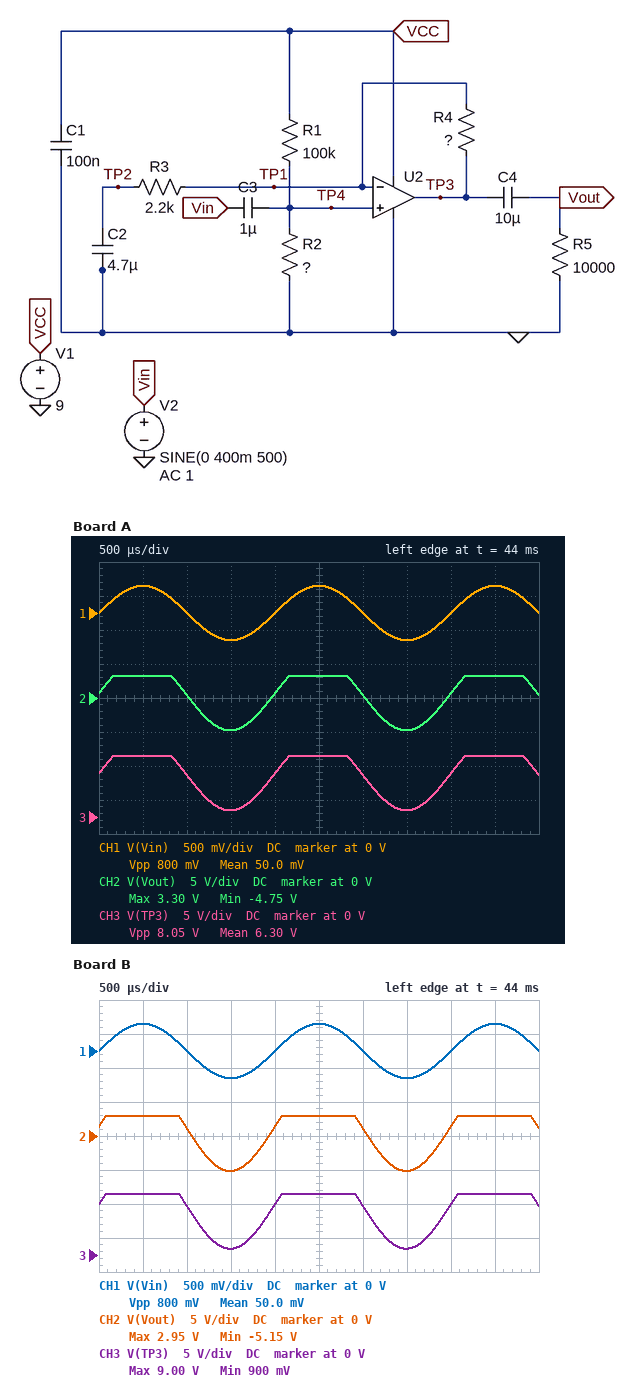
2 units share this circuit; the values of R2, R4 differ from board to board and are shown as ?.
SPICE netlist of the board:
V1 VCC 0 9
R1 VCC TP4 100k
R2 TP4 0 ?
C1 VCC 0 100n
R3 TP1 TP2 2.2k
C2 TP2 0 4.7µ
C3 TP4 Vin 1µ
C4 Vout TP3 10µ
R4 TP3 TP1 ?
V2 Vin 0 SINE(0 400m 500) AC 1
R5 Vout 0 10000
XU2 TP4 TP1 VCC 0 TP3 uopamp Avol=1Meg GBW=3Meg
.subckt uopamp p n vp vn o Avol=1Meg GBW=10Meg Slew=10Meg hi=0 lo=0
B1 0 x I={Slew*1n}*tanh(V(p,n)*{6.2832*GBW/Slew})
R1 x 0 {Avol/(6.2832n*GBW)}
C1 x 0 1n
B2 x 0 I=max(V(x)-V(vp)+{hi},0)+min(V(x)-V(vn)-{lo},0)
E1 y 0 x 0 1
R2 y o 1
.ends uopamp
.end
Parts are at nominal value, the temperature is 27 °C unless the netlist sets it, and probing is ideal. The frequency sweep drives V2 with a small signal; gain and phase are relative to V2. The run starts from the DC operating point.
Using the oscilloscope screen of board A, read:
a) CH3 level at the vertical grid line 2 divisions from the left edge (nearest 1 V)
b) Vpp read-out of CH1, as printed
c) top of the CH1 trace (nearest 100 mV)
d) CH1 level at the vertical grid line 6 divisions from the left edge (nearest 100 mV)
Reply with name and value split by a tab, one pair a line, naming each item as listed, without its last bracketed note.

CH3 level at the vertical grid line 2 divisions from the left edge	6 V
Vpp read-out of CH1, as printed	800 mV
top of the CH1 trace	400 mV
CH1 level at the vertical grid line 6 divisions from the left edge	0 V
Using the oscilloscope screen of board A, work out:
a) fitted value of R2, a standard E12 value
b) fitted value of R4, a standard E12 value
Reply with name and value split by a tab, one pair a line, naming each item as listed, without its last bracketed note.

fitted value of R2, a standard E12 value	180 kΩ
fitted value of R4, a standard E12 value	27 kΩ
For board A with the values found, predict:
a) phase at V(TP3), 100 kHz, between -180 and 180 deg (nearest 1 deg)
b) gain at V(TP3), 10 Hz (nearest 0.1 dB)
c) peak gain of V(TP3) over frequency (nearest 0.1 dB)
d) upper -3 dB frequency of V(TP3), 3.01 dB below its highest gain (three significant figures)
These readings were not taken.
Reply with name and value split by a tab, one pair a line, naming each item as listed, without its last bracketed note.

phase at V(TP3), 100 kHz, between -180 and 180 deg	-24 deg
gain at V(TP3), 10 Hz	17.0 dB
peak gain of V(TP3) over frequency	22.5 dB
upper -3 dB frequency of V(TP3), 3.01 dB below its highest gain	226 kHz
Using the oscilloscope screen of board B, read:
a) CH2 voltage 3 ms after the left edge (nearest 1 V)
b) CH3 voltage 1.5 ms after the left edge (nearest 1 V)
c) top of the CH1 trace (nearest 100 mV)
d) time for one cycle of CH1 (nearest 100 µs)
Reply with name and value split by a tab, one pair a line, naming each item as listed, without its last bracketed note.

CH2 voltage 3 ms after the left edge	1 V
CH3 voltage 1.5 ms after the left edge	1 V
top of the CH1 trace	400 mV
time for one cycle of CH1	2.0 ms
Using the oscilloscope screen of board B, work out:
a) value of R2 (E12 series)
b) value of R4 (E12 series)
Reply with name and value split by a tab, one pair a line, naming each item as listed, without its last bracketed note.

value of R2	220 kΩ
value of R4	33 kΩ
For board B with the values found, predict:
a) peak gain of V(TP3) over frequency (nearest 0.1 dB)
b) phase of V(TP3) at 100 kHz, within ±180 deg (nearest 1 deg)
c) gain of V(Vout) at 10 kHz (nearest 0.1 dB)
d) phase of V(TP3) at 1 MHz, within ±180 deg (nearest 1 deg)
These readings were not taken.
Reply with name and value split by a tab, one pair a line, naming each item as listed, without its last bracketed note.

peak gain of V(TP3) over frequency	24.1 dB
phase of V(TP3) at 100 kHz, within ±180 deg	-28 deg
gain of V(Vout) at 10 kHz	24.1 dB
phase of V(TP3) at 1 MHz, within ±180 deg	-79 deg
